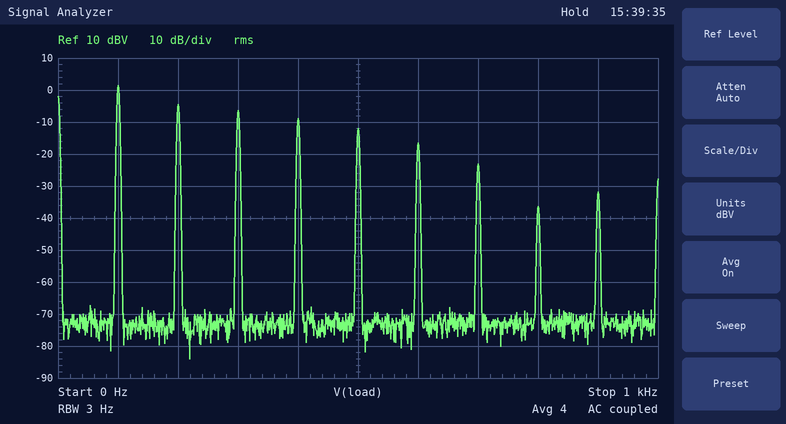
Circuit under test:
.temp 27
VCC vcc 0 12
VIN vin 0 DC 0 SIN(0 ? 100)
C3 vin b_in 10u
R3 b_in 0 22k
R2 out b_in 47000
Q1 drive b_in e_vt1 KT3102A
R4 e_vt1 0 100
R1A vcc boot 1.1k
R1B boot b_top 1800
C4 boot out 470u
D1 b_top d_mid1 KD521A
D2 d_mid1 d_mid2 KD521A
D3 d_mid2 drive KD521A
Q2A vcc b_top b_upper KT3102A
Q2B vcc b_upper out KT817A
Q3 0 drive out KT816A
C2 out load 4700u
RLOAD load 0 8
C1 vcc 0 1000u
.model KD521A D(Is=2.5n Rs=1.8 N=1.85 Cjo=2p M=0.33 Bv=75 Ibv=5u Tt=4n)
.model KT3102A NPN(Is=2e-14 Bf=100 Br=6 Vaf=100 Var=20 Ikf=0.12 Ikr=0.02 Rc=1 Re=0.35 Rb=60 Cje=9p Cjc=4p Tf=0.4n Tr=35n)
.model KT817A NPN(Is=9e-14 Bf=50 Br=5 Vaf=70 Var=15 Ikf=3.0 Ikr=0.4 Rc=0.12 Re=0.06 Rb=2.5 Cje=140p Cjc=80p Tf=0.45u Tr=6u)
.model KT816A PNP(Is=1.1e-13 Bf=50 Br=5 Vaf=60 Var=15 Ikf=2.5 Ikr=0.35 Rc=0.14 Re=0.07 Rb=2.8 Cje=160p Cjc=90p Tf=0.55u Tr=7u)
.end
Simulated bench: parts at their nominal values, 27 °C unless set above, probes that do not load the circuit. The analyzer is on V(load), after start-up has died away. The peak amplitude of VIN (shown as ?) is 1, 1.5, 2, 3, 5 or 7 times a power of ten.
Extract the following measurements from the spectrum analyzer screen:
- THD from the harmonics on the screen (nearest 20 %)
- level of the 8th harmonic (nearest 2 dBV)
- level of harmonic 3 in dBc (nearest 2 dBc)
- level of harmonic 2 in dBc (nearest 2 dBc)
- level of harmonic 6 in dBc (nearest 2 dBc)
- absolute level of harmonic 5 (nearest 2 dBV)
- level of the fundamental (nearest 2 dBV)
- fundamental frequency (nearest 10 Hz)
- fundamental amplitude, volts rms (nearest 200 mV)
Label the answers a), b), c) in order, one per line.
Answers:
a) 80 %
b) -36 dBV
c) -8 dBc
d) -6 dBc
e) -18 dBc
f) -12 dBV
g) 2 dBV
h) 100 Hz
i) 1.2 V
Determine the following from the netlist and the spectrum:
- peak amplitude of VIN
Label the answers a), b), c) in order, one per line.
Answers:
a) 200 mV
